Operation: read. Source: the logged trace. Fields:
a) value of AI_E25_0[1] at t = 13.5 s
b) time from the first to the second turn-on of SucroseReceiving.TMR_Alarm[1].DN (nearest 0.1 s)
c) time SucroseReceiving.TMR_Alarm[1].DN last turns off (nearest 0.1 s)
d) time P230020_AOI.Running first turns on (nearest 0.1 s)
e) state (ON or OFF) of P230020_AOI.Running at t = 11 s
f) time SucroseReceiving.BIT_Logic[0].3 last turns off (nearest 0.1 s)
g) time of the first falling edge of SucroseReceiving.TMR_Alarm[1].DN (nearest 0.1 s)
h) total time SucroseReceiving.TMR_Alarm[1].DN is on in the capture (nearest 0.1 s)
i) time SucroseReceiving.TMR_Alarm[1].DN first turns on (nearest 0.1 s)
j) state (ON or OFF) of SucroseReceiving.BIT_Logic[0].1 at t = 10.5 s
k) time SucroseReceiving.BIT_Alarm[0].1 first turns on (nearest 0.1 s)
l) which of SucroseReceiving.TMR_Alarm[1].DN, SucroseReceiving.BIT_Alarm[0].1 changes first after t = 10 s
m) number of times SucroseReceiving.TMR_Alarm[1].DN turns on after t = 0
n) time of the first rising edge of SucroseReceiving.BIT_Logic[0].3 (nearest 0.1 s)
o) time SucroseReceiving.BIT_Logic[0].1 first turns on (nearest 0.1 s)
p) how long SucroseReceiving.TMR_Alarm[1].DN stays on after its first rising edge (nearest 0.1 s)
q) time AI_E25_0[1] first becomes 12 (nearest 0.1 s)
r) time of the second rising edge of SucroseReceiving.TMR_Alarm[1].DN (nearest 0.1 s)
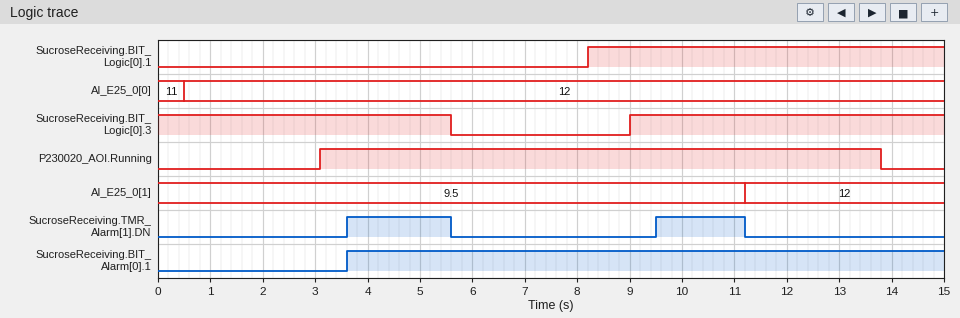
12
5.9 s
11.2 s
3.1 s
ON
5.6 s
5.6 s
3.7 s
3.6 s
ON
3.6 s
SucroseReceiving.TMR_Alarm[1].DN
2
9.0 s
8.2 s
2.0 s
11.2 s
9.5 s
